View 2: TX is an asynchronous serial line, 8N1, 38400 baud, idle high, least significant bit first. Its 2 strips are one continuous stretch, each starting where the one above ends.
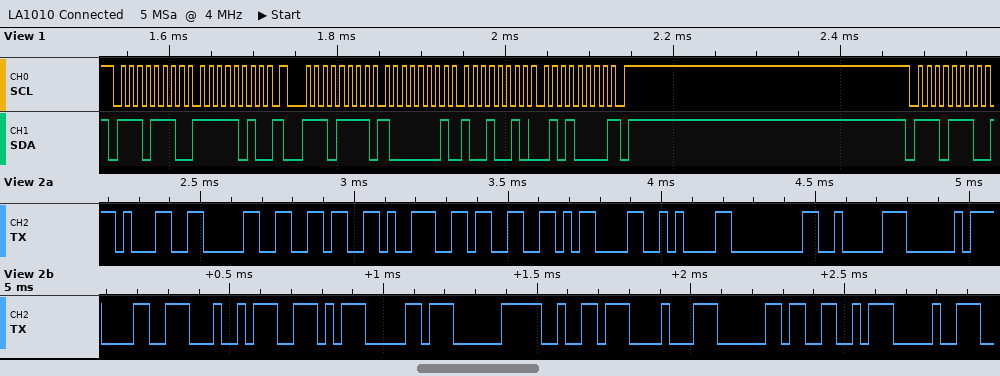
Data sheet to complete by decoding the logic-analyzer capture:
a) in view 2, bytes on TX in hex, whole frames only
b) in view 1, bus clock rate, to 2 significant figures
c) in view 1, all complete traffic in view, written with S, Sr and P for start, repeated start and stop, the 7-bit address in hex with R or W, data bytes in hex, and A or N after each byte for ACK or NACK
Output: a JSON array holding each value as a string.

["31 30 36 39 33 0D 0A 00 82 A0 98 A4 AE B0 E0 B2 88 60 A6 90", "100 kHz", "S 77W A FA A Sr 77R A 81 A 92 A 50 N P S 77W A"]
